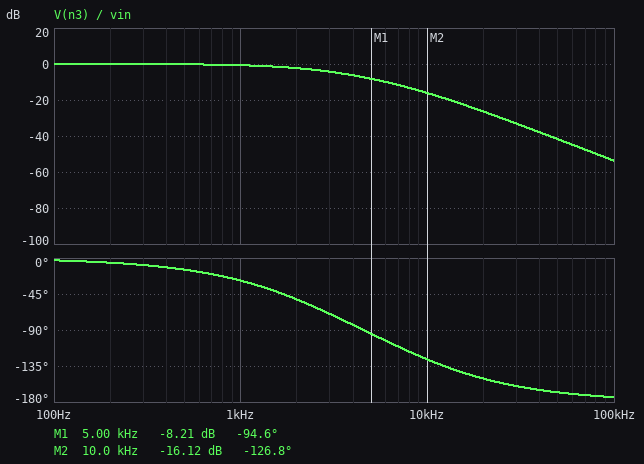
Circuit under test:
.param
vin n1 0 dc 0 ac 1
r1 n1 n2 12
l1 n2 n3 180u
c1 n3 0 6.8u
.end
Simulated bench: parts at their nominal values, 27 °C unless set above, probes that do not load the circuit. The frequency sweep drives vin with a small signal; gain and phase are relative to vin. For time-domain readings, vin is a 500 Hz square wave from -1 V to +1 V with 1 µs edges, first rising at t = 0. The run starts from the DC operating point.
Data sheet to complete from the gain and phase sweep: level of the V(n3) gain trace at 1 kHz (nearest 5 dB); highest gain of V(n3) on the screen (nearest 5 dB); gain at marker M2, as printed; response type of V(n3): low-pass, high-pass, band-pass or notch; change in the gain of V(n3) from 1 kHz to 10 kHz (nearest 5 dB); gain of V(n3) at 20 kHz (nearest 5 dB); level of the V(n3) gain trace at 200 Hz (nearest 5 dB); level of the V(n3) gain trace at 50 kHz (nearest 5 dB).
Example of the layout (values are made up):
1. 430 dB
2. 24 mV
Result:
1. 0 dB
2. 0 dB
3. -16.12 dB
4. low-pass
5. -15 dB
6. -25 dB
7. 0 dB
8. -40 dB
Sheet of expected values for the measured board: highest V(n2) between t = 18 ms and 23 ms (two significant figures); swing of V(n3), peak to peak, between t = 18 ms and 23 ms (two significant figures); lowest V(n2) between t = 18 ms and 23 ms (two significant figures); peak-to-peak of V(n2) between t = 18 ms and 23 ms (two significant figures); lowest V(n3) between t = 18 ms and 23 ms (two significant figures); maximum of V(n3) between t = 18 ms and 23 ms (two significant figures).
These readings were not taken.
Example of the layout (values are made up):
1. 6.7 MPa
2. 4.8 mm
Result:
1. 1.0 V
2. 2.0 V
3. -1.0 V
4. 2.0 V
5. -1.0 V
6. 1.0 V
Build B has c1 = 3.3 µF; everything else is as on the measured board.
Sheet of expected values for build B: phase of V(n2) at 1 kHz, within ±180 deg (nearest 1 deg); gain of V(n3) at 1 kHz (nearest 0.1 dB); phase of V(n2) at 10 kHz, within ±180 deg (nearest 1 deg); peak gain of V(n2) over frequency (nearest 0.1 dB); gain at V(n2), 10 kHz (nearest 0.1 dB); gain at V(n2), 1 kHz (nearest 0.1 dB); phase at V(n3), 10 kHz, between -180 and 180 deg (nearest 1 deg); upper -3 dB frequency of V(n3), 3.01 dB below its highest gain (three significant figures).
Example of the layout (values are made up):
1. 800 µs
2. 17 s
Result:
1. -14 deg
2. -0.1 dB
3. 62 deg
4. 0 dB
5. -6.5 dB
6. -0.3 dB
7. -118 deg
8. 5.58 kHz
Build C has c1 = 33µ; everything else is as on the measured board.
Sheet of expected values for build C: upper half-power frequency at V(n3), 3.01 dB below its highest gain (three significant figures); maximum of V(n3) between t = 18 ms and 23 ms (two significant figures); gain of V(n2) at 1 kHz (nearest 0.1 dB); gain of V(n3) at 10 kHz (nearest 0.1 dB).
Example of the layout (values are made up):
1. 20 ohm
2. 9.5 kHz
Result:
1. 418 Hz
2. 860 mV
3. -10.6 dB
4. -30.5 dB
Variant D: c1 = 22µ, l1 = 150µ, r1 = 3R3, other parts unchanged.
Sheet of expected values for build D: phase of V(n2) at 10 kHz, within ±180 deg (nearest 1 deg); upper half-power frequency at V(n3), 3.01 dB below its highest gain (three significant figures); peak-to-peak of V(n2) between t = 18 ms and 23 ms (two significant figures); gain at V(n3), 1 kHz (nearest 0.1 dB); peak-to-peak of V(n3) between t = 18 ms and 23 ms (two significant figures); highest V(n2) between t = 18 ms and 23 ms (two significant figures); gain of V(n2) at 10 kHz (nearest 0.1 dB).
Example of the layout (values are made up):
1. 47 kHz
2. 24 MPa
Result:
1. 21 deg
2. 3.01 kHz
3. 2.2 V
4. 0.2 dB
5. 2.3 V
6. 1.1 V
7. -0.6 dB
